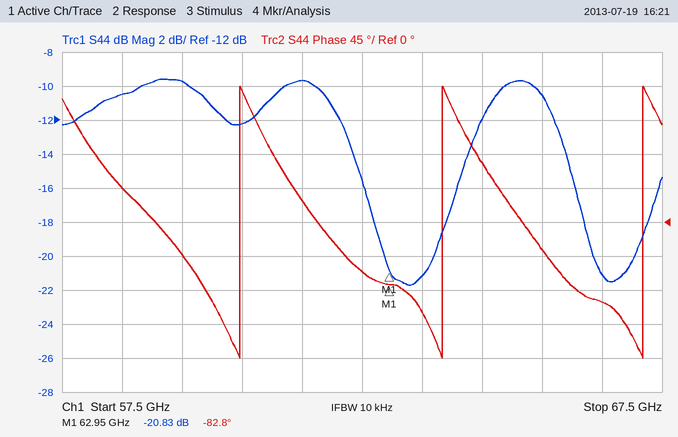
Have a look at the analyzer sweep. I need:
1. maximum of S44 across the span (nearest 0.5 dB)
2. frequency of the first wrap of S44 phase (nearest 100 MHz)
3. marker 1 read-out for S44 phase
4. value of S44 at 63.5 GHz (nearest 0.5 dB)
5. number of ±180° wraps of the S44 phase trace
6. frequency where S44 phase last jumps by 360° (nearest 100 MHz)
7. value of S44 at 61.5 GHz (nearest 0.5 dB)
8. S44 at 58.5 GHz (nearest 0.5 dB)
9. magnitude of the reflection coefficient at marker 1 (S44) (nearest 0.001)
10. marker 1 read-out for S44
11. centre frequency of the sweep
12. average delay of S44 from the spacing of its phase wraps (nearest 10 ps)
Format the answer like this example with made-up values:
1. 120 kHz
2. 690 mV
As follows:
1. -9.5 dB
2. 60.5 GHz
3. -82.8°
4. -21.0 dB
5. 3
6. 67.2 GHz
7. -9.5 dB
8. -10.5 dB
9. 0.091
10. -20.83 dB
11. 62.5 GHz
12. 300 ps
